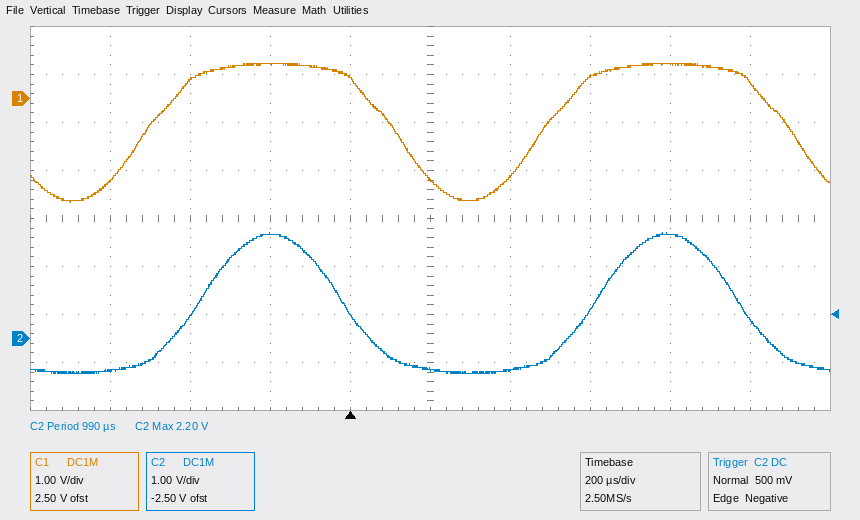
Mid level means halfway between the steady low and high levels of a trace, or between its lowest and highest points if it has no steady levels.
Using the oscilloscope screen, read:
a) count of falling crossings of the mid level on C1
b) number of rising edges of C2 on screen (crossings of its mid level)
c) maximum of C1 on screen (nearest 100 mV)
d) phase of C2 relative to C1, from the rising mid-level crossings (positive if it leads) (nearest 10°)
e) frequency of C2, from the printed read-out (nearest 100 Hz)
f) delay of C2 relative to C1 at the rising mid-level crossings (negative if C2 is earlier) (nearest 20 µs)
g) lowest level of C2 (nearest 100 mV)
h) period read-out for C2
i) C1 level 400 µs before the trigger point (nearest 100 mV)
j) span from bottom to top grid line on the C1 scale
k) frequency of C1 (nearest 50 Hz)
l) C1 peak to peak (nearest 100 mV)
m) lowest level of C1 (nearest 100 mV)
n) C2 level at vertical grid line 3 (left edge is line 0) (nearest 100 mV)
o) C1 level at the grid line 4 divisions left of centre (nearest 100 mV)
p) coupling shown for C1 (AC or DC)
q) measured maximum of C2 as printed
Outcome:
2
2
700 mV
-50°
1.0 kHz
+140 µs
-700 mV
990 µs
400 mV
8 V
1.00 kHz
2.9 V
-2.2 V
2.2 V
-1.7 V
DC
2.20 V
